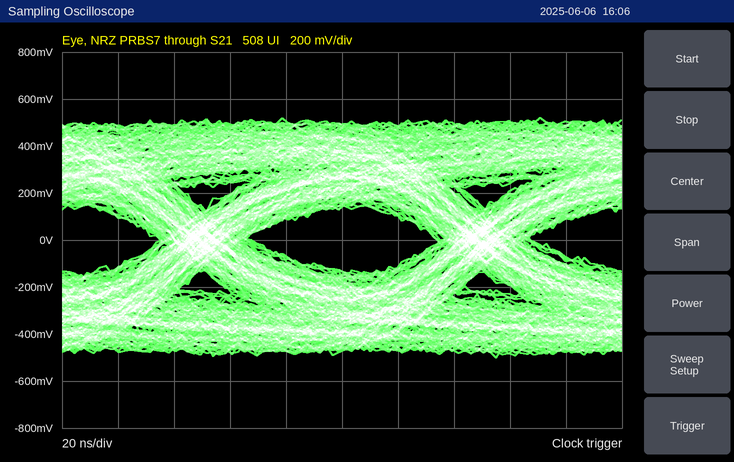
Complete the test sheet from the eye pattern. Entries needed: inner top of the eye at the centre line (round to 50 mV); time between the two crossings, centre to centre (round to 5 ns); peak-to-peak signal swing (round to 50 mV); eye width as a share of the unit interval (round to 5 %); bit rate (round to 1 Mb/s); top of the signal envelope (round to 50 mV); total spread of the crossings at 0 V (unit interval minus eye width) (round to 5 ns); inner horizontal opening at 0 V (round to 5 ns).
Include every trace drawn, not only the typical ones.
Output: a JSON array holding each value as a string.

["150 mV", "100 ns", "1.00 V", "65 %", "10 Mb/s", "500 mV", "35 ns", "65 ns"]
